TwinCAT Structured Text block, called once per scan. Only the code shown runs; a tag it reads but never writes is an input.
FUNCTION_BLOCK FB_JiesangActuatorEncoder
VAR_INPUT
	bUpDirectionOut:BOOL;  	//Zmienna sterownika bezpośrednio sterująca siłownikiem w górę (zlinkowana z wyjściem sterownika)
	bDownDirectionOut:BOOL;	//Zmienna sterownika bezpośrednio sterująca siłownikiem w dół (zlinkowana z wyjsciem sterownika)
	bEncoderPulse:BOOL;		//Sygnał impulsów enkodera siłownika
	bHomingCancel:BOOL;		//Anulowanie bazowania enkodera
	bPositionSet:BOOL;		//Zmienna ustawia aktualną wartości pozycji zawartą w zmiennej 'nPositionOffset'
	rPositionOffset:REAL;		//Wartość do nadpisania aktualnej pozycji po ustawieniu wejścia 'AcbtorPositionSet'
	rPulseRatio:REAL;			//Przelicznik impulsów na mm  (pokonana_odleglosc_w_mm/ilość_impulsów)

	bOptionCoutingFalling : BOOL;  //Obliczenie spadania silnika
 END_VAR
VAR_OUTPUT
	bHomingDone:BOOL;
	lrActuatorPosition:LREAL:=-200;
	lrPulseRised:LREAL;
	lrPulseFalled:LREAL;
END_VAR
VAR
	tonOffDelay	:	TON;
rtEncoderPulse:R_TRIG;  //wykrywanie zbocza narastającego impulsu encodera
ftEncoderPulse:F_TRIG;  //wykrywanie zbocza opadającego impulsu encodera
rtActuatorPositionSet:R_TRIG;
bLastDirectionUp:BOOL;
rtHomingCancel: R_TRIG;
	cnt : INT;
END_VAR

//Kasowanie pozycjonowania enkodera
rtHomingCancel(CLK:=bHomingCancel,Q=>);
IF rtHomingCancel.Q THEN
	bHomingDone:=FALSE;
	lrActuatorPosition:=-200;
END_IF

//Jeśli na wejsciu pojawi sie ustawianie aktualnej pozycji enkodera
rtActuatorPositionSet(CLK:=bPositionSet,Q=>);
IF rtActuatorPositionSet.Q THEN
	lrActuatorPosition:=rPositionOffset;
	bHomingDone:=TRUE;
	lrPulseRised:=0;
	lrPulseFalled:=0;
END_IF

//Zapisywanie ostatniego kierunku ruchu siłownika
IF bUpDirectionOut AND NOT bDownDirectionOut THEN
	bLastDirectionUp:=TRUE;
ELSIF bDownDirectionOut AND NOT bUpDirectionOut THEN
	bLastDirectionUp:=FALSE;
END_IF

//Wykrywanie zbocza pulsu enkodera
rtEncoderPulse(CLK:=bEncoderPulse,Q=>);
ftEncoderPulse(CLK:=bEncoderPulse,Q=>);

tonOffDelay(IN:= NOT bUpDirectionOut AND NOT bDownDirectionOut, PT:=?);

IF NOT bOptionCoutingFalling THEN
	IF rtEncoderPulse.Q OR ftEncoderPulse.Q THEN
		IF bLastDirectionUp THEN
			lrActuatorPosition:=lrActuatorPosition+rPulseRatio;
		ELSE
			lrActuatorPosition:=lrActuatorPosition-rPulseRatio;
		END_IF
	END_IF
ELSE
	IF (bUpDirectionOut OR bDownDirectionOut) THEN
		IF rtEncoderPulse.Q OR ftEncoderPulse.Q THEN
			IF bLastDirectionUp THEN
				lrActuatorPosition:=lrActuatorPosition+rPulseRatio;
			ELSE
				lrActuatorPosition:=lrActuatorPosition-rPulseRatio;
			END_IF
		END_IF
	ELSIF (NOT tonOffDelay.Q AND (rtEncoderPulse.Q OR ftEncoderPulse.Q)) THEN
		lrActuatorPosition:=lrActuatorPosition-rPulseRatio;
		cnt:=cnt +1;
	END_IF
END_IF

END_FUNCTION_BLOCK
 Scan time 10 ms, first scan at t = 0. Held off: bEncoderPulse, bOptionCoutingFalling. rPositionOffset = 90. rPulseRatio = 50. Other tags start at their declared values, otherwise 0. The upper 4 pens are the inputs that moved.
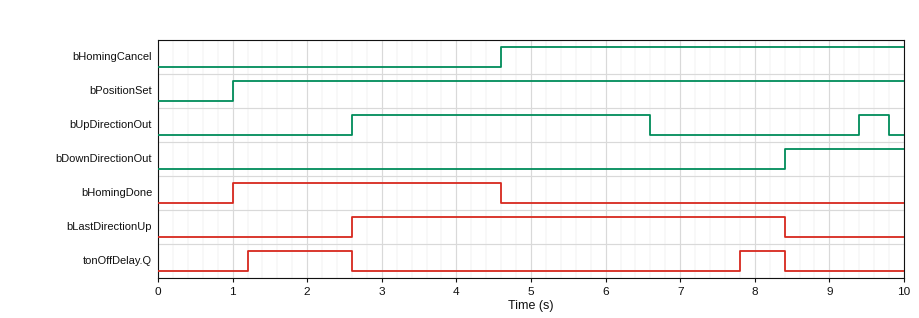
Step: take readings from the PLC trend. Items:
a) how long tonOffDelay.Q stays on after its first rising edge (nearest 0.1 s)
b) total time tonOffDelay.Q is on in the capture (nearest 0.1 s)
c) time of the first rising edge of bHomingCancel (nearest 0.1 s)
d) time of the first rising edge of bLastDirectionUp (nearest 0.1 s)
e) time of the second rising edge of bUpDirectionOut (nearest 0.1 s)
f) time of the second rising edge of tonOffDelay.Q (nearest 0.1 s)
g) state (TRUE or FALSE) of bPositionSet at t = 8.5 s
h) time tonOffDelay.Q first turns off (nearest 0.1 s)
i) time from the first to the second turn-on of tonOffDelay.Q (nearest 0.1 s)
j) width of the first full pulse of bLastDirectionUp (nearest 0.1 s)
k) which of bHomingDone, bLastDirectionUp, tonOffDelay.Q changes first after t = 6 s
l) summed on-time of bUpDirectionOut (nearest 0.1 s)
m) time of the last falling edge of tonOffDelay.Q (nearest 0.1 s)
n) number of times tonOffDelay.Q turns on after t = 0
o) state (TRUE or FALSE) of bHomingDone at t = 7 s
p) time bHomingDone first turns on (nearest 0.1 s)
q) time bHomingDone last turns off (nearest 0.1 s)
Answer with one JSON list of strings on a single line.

["1.4 s", "2.0 s", "4.6 s", "2.6 s", "9.4 s", "7.8 s", "TRUE", "2.6 s", "6.6 s", "5.8 s", "tonOffDelay.Q", "4.4 s", "8.4 s", "2", "FALSE", "1.0 s", "4.6 s"]
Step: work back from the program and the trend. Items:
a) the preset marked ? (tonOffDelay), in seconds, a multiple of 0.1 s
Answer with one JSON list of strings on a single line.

["1.2 s"]
